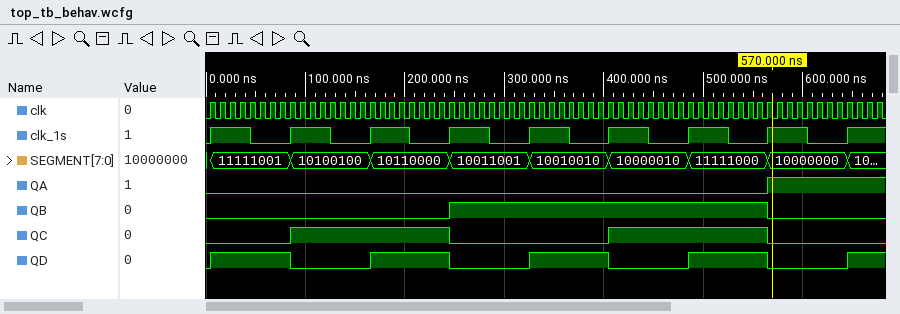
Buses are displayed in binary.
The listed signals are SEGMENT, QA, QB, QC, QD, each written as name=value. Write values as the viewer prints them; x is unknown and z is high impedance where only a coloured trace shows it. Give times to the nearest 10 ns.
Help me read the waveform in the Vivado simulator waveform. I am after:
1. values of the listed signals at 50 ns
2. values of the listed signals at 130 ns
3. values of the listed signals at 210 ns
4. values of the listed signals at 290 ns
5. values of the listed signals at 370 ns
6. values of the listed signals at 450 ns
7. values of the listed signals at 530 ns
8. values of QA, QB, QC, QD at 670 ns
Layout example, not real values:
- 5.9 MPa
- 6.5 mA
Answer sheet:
- SEGMENT=11111001, QA=0, QB=0, QC=0, QD=1
- SEGMENT=10100100, QA=0, QB=0, QC=1, QD=0
- SEGMENT=10110000, QA=0, QB=0, QC=1, QD=1
- SEGMENT=10011001, QA=0, QB=1, QC=0, QD=0
- SEGMENT=10010010, QA=0, QB=1, QC=0, QD=1
- SEGMENT=10000010, QA=0, QB=1, QC=1, QD=0
- SEGMENT=11111000, QA=0, QB=1, QC=1, QD=1
- QA=1, QB=0, QC=0, QD=1
